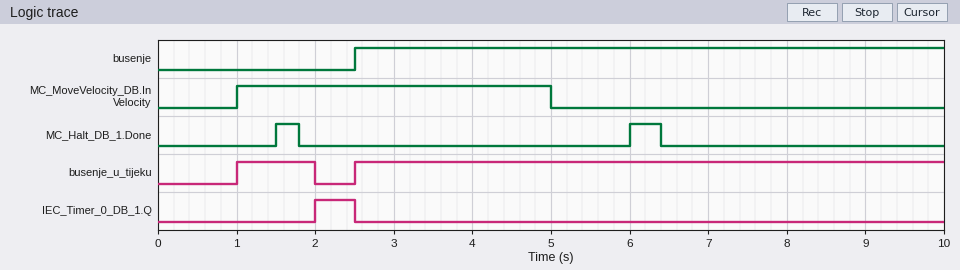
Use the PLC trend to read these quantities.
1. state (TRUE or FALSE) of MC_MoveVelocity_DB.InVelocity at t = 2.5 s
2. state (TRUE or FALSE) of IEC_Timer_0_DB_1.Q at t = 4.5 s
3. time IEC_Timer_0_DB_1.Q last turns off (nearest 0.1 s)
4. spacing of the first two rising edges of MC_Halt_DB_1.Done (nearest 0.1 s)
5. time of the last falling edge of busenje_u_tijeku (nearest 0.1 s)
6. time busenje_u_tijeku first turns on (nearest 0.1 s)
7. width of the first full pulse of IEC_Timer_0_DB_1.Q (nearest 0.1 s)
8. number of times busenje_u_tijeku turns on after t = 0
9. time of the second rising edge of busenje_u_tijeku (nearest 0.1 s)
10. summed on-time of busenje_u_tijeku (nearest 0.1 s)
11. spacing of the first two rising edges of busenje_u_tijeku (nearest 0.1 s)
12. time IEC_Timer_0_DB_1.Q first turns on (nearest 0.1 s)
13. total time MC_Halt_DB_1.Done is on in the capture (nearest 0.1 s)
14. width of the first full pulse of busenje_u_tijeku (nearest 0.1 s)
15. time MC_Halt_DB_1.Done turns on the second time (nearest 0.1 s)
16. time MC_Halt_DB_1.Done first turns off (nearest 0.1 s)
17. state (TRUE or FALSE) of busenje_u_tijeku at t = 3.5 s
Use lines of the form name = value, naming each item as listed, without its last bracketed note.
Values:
state (TRUE or FALSE) of MC_MoveVelocity_DB.InVelocity at t = 2.5 s = TRUE
state (TRUE or FALSE) of IEC_Timer_0_DB_1.Q at t = 4.5 s = FALSE
time IEC_Timer_0_DB_1.Q last turns off = 2.5 s
spacing of the first two rising edges of MC_Halt_DB_1.Done = 4.5 s
time of the last falling edge of busenje_u_tijeku = 2.0 s
time busenje_u_tijeku first turns on = 1.0 s
width of the first full pulse of IEC_Timer_0_DB_1.Q = 0.5 s
number of times busenje_u_tijeku turns on after t = 0 = 2
time of the second rising edge of busenje_u_tijeku = 2.5 s
summed on-time of busenje_u_tijeku = 8.5 s
spacing of the first two rising edges of busenje_u_tijeku = 1.5 s
time IEC_Timer_0_DB_1.Q first turns on = 2.0 s
total time MC_Halt_DB_1.Done is on in the capture = 0.7 s
width of the first full pulse of busenje_u_tijeku = 1.0 s
time MC_Halt_DB_1.Done turns on the second time = 6.0 s
time MC_Halt_DB_1.Done first turns off = 1.8 s
state (TRUE or FALSE) of busenje_u_tijeku at t = 3.5 s = TRUE
